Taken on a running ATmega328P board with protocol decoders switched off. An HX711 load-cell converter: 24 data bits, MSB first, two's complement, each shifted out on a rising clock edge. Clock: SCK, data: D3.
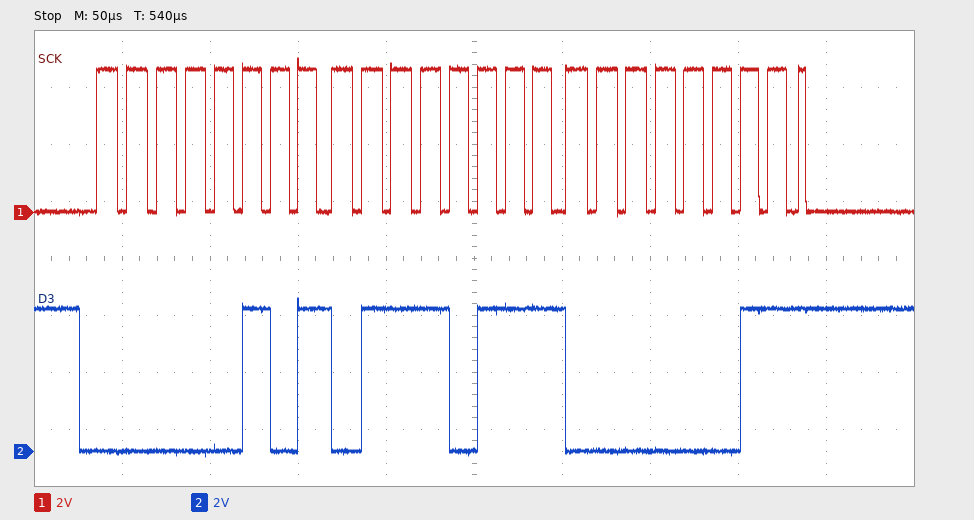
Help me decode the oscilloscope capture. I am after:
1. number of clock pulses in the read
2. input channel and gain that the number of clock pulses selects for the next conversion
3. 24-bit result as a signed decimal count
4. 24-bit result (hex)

25
channel A, gain 128
358147
0x057703
